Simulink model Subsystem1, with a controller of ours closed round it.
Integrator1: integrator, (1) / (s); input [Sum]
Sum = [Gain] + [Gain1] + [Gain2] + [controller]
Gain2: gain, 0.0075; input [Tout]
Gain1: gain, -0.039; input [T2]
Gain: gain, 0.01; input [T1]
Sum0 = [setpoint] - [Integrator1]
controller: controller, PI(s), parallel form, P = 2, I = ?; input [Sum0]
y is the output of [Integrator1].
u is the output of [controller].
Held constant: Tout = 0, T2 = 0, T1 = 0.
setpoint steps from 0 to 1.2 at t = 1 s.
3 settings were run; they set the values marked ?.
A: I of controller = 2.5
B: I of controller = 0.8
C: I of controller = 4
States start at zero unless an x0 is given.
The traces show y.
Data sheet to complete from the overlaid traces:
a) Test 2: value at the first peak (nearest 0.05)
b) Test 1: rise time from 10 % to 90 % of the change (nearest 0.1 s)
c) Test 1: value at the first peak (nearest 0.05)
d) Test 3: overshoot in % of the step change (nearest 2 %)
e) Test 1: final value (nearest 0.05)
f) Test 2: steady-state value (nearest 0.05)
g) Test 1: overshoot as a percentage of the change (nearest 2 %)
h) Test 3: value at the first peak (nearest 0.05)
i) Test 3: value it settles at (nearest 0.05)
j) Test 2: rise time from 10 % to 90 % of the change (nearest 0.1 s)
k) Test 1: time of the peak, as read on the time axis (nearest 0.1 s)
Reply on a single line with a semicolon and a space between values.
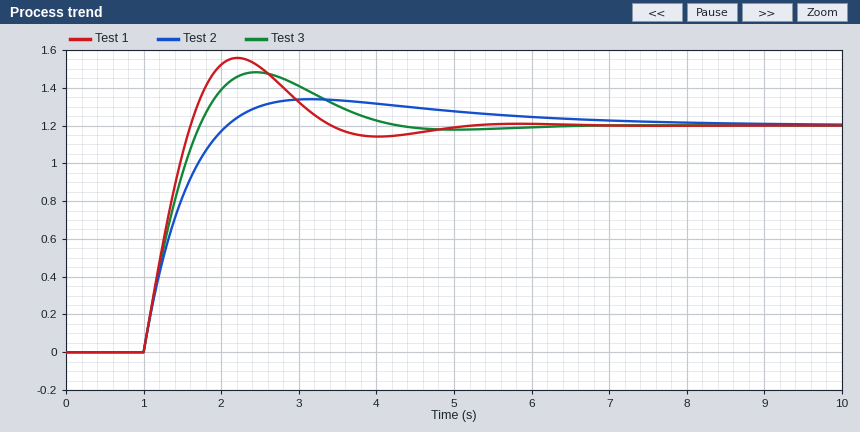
1.35; 0.5 s; 1.55; 24 %; 1.20; 1.20; 30 %; 1.50; 1.20; 0.8 s; 2.2 s
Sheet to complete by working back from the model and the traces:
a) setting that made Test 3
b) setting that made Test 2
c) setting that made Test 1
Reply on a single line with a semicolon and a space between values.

A; B; C
